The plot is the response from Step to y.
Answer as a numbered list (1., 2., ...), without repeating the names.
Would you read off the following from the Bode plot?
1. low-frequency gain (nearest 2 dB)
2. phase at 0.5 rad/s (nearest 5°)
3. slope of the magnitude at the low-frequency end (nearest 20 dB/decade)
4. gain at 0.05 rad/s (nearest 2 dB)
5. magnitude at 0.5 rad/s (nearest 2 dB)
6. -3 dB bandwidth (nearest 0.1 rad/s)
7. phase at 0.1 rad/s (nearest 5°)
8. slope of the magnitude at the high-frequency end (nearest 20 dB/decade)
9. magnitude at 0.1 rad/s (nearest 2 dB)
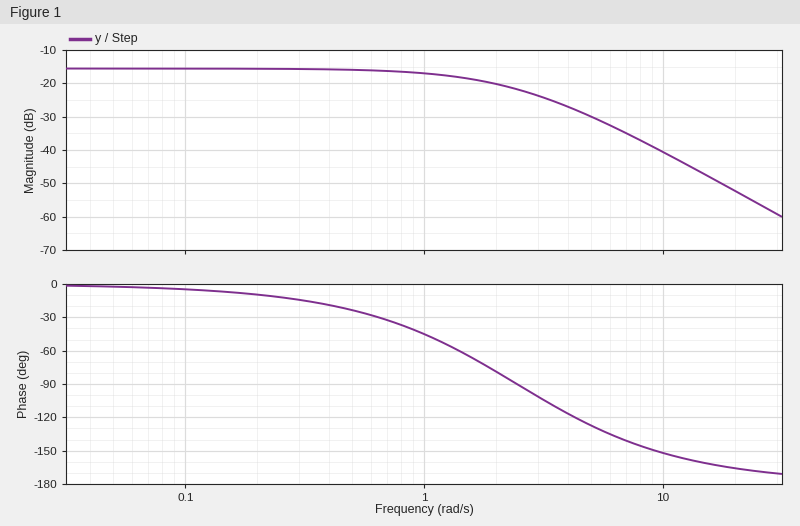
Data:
1. -16 dB
2. -25°
3. 0 dB/decade
4. -16 dB
5. -16 dB
6. 1.5 rad/s
7. -5°
8. -40 dB/decade
9. -16 dB
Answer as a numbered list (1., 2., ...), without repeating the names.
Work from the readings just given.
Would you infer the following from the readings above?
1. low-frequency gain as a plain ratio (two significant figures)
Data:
1. 0.16
